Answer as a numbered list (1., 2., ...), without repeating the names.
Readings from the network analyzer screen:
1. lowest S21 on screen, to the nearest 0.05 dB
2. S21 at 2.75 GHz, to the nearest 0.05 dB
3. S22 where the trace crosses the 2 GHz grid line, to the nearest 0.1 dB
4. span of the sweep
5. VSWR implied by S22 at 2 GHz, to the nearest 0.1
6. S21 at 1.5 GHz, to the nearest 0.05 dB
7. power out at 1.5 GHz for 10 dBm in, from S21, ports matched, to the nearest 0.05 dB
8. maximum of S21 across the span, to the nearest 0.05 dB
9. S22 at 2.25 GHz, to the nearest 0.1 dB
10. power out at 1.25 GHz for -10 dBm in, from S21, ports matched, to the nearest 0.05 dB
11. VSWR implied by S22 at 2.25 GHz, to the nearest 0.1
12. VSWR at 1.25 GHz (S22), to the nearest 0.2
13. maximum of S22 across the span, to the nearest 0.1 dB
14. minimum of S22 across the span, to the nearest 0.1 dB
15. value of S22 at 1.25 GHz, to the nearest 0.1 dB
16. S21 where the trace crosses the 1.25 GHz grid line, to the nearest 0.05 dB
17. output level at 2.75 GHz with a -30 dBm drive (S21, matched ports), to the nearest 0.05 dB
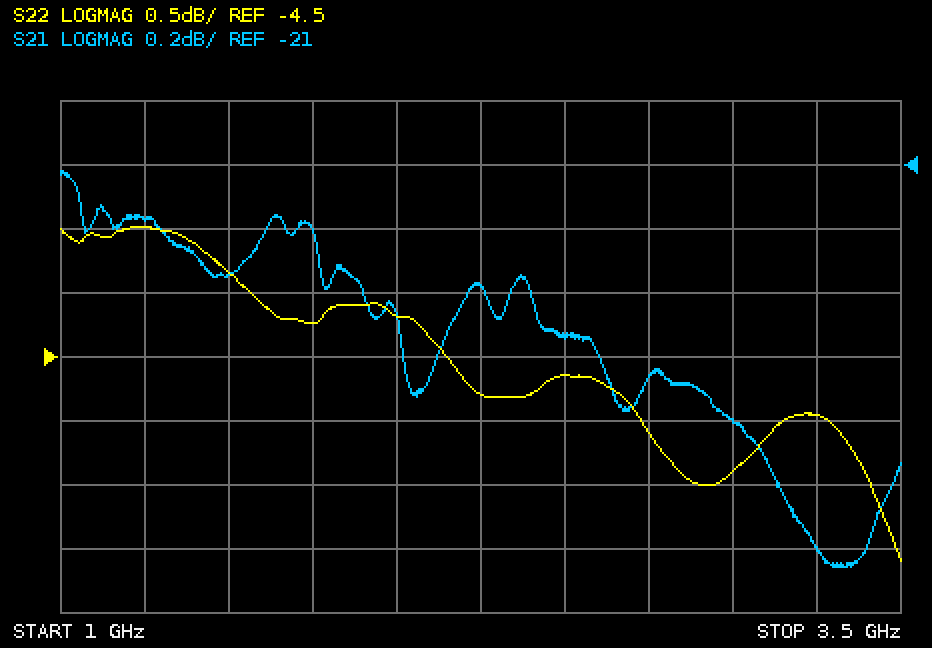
1. -22.25 dB
2. -21.65 dB
3. -4.2 dB
4. 2.5 GHz
5. 4.2
6. -21.35 dB
7. -11.35 dBm
8. -21.00 dB
9. -4.8 dB
10. -31.15 dBm
11. 3.7
12. 5.0
13. -3.5 dB
14. -6.1 dB
15. -3.5 dB
16. -21.15 dB
17. -51.65 dBm
